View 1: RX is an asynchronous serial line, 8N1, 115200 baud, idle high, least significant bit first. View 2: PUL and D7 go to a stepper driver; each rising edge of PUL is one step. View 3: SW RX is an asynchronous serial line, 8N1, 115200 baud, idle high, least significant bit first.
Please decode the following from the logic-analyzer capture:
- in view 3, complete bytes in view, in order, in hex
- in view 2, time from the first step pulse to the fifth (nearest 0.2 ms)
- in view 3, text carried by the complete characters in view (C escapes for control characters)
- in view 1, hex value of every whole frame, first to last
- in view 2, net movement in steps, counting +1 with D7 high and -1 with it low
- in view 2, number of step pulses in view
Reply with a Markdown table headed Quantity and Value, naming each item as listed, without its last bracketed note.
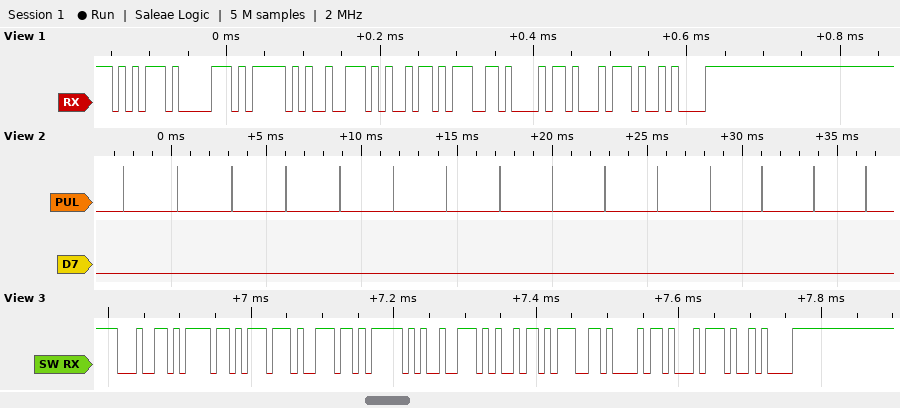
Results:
| Quantity | Value |
|---|---|
| in view 3, complete bytes in view, in order, in hex | 64 6F 77 6E 5F 72 69 67 68 74 0A |
| in view 2, time from the first step pulse to the fifth | 11.4 ms |
| in view 3, text carried by the complete characters in view | "down_right\n" |
| in view 1, hex value of every whole frame, first to last | 75 70 5F 72 69 67 68 74 0A |
| in view 2, net movement in steps, counting +1 with D7 high and -1 with it low | -15 |
| in view 2, number of step pulses in view | 15 |
